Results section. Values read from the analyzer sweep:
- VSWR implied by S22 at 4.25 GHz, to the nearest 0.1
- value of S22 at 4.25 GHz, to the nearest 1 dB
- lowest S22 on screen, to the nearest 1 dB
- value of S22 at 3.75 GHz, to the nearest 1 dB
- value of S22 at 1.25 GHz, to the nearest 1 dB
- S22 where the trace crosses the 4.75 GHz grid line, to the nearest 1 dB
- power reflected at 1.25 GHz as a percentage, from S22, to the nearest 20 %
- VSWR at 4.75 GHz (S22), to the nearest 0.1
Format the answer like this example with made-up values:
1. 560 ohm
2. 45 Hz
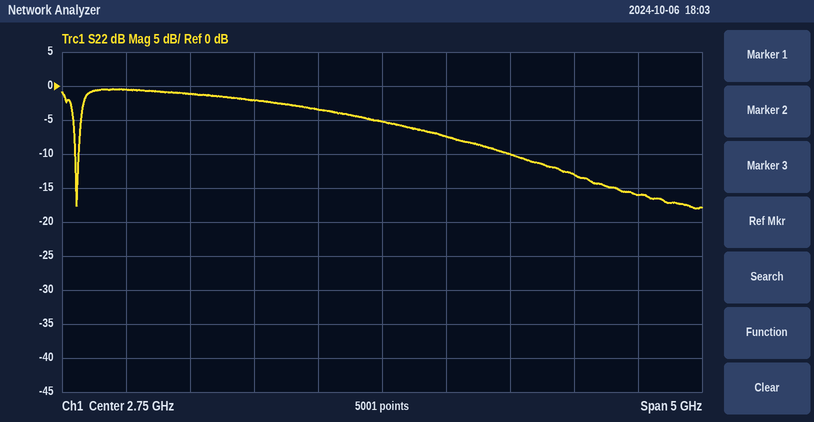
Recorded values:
1. 1.6
2. -13 dB
3. -18 dB
4. -10 dB
5. -1 dB
6. -16 dB
7. 80 %
8. 1.4
